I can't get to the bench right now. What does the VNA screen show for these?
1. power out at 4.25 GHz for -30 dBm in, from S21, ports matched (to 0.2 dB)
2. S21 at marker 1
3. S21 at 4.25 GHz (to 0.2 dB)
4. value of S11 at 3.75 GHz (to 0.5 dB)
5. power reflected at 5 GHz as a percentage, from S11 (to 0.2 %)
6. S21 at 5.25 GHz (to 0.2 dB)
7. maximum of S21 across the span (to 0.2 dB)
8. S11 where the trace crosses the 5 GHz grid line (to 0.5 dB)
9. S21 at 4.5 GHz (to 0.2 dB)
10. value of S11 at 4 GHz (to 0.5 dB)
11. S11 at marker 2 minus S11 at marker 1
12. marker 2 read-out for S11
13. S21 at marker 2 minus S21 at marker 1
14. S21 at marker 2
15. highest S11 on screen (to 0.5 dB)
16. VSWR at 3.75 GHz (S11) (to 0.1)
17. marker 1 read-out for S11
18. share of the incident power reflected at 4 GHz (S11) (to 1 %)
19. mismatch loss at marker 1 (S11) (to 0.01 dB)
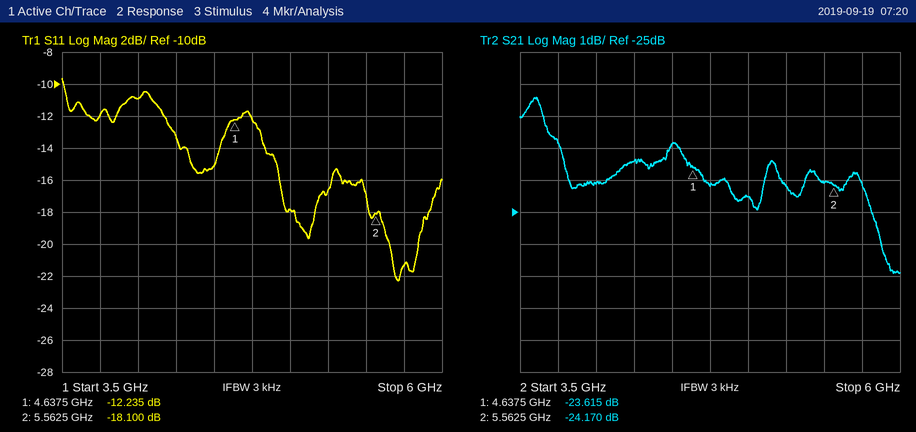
-53.4 dBm
-23.615 dB
-23.4 dB
-12.0 dB
1.6 %
-24.2 dB
-21.4 dB
-18.0 dB
-22.8 dB
-11.0 dB
-5.865 dB
-18.100 dB
-0.555 dB
-24.170 dB
-9.5 dB
1.7
-12.235 dB
8 %
0.27 dB
